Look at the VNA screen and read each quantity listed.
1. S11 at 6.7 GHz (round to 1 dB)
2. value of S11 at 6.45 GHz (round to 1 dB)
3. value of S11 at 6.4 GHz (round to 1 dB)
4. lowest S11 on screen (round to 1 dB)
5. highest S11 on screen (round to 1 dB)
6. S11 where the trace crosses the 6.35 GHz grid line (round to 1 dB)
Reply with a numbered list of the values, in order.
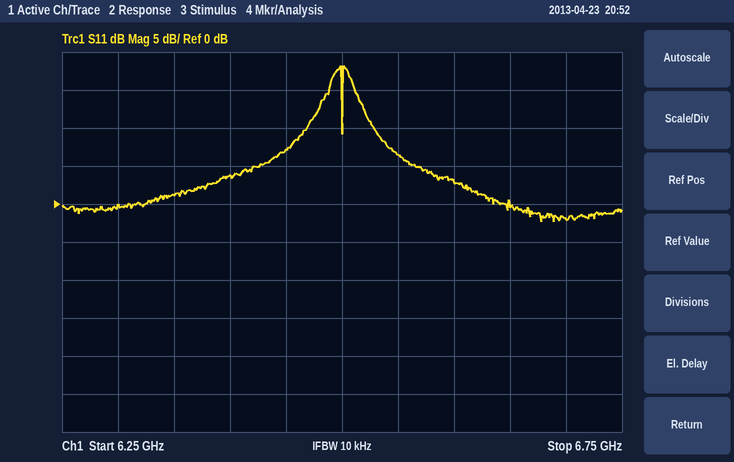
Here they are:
1. -2 dB
2. 7 dB
3. 4 dB
4. -2 dB
5. 18 dB
6. 1 dB
